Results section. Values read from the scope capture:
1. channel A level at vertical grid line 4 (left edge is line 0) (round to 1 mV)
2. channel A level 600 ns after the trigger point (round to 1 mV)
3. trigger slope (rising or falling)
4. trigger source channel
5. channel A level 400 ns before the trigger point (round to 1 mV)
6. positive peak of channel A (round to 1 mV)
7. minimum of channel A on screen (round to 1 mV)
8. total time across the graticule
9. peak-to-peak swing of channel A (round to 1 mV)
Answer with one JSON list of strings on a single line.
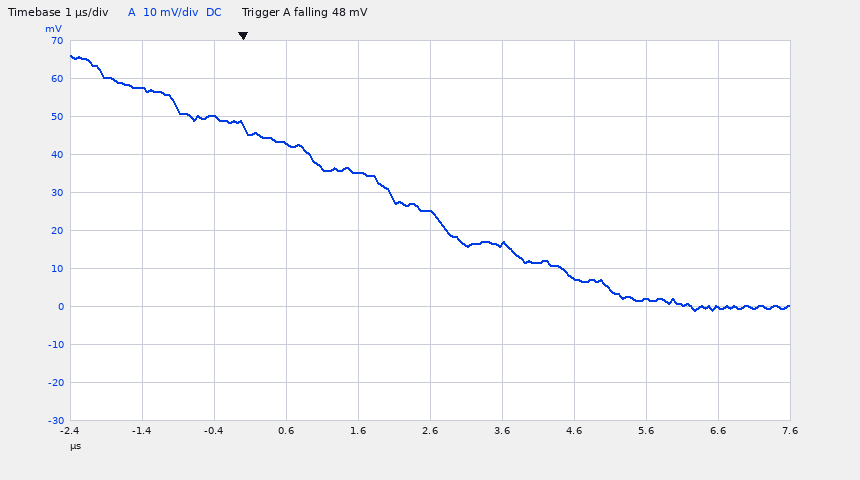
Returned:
["35 mV", "43 mV", "falling", "channel A", "50 mV", "66 mV", "-1 mV", "10 µs", "67 mV"]
